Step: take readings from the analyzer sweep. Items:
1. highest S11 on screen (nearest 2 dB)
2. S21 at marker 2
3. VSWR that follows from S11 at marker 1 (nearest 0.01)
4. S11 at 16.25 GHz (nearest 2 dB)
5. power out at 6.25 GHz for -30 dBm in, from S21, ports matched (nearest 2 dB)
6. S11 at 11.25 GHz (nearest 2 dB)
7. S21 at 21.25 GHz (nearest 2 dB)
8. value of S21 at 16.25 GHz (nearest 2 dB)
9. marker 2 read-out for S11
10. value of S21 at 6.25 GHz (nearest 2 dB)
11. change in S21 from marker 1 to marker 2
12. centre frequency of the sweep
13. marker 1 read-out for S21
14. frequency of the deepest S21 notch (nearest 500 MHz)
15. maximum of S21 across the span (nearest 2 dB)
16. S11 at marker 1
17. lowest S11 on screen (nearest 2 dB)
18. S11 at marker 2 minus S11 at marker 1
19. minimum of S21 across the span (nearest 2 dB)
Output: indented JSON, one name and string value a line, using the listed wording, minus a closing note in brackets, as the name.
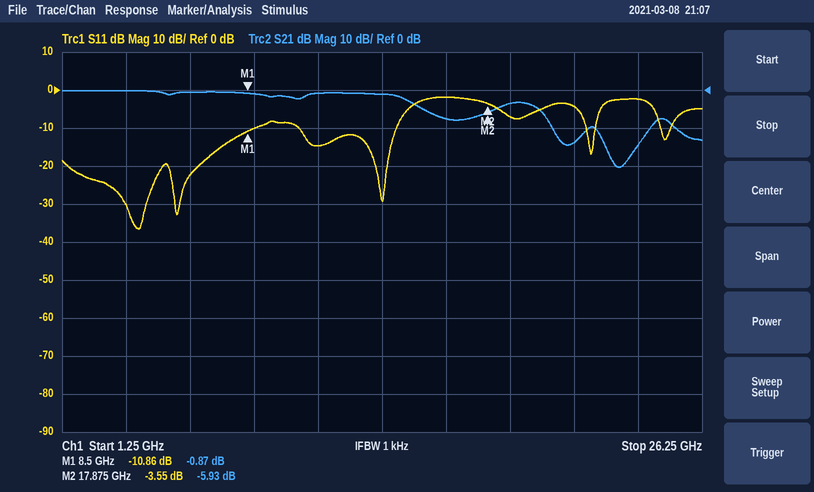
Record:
{
  "highest S11 on screen": "-2 dB",
  "S21 at marker 2": "-5.93 dB",
  "VSWR that follows from S11 at marker 1": "1.80",
  "S11 at 16.25 GHz": "-2 dB",
  "power out at 6.25 GHz for -30 dBm in, from S21, ports matched": "-30 dBm",
  "S11 at 11.25 GHz": "-14 dB",
  "S21 at 21.25 GHz": "-14 dB",
  "value of S21 at 16.25 GHz": "-8 dB",
  "marker 2 read-out for S11": "-3.55 dB",
  "value of S21 at 6.25 GHz": "0 dB",
  "change in S21 from marker 1 to marker 2": "-5.06 dB",
  "centre frequency of the sweep": "13.75 GHz",
  "marker 1 read-out for S21": "-0.87 dB",
  "frequency of the deepest S21 notch": "23.0 GHz",
  "maximum of S21 across the span": "0 dB",
  "S11 at marker 1": "-10.86 dB",
  "lowest S11 on screen": "-36 dB",
  "S11 at marker 2 minus S11 at marker 1": "7.31 dB",
  "minimum of S21 across the span": "-20 dB"
}
